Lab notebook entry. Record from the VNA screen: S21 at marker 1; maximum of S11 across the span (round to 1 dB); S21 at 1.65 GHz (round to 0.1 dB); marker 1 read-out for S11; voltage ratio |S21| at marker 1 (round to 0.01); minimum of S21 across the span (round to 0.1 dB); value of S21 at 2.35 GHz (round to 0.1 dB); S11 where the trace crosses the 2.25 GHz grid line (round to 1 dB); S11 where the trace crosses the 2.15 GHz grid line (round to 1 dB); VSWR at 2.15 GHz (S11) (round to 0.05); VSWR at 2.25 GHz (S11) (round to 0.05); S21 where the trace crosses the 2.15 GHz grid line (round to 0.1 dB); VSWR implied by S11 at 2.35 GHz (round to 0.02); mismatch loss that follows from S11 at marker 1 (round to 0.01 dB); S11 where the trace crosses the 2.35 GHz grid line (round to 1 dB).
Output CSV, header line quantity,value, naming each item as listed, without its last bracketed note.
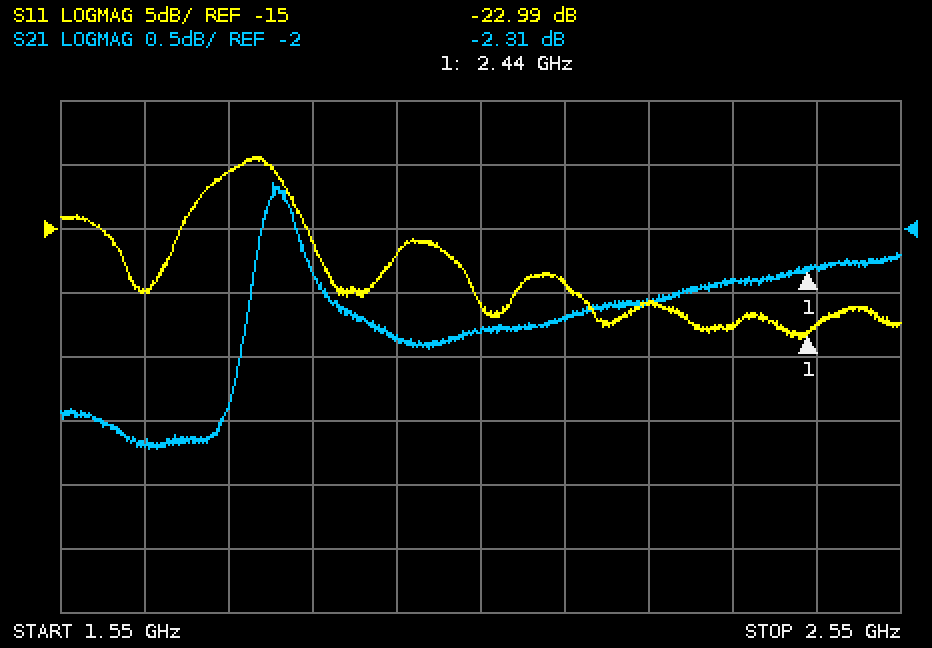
quantity,value
S21 at marker 1,-2.31 dB
maximum of S11 across the span,-9 dB
S21 at 1.65 GHz,-3.7 dB
marker 1 read-out for S11,-22.99 dB
voltage ratio |S21| at marker 1,0.77
minimum of S21 across the span,-3.7 dB
value of S21 at 2.35 GHz,-2.4 dB
S11 where the trace crosses the 2.25 GHz grid line,-21 dB
S11 where the trace crosses the 2.15 GHz grid line,-19 dB
VSWR at 2.15 GHz (S11),1.25
VSWR at 2.25 GHz (S11),1.20
S21 where the trace crosses the 2.15 GHz grid line,-2.7 dB
VSWR implied by S11 at 2.35 GHz,1.16
mismatch loss that follows from S11 at marker 1,0.02 dB
S11 where the trace crosses the 2.35 GHz grid line,-23 dB
